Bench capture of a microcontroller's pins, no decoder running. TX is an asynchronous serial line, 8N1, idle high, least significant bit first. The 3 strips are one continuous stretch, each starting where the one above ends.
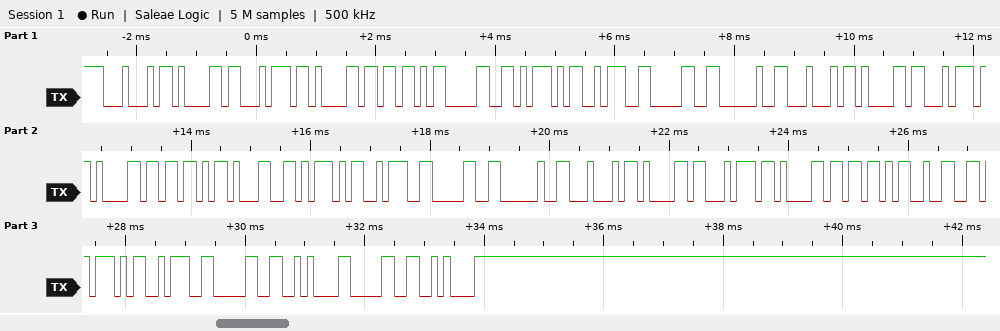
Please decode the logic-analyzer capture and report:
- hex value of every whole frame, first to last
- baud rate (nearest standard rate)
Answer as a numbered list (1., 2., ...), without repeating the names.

1. 44 61 74 61 5B 30 5D 3A 30 20 44 61 74 61 5B 31 5D 3A 30 20 44 61 74 61 5B 32 5D 3A 30 0A 30 0A
2. 9600 baud
